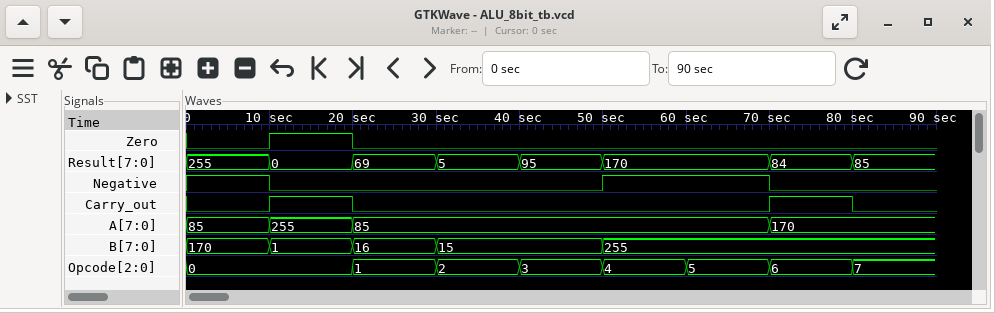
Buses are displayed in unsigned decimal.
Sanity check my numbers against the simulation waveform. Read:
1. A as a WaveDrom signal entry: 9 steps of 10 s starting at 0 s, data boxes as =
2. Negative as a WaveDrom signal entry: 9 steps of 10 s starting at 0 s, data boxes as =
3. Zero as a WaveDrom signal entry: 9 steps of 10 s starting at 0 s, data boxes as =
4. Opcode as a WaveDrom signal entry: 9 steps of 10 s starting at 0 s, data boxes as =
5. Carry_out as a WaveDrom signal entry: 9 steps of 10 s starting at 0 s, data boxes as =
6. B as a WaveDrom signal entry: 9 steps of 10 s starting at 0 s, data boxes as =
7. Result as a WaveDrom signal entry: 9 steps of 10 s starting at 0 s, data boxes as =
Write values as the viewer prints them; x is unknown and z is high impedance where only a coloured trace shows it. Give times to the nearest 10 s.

{name: 'A', wave: '===....=.', data: '85 255 85 170'}
{name: 'Negative', wave: '10...1.0.'}
{name: 'Zero', wave: '010......'}
{name: 'Opcode', wave: '=.=======', data: '0 1 2 3 4 5 6 7'}
{name: 'Carry_out', wave: '010....10'}
{name: 'B', wave: '====.=...', data: '170 1 16 15 255'}
{name: 'Result', wave: '======.==', data: '255 0 69 5 95 170 84 85'}
